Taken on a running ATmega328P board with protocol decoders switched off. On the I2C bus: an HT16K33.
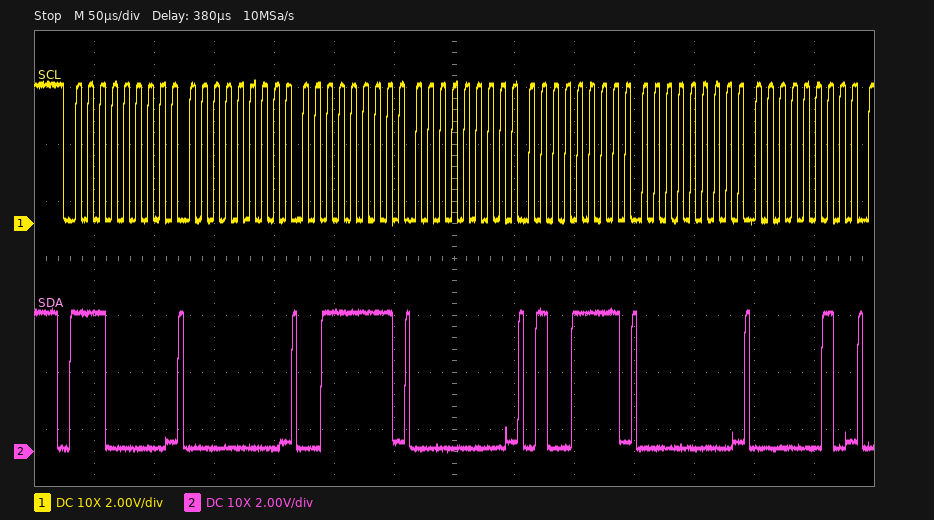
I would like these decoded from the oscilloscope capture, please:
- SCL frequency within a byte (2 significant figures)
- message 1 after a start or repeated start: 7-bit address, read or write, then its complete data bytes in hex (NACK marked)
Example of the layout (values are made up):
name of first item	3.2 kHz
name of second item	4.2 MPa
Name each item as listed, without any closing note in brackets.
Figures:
SCL frequency within a byte	100 kHz
message 1 after a start or repeated start: 7-bit address, read or write, then its complete data bytes in hex	0x70 write: 00 3F 00 4F 00 02
